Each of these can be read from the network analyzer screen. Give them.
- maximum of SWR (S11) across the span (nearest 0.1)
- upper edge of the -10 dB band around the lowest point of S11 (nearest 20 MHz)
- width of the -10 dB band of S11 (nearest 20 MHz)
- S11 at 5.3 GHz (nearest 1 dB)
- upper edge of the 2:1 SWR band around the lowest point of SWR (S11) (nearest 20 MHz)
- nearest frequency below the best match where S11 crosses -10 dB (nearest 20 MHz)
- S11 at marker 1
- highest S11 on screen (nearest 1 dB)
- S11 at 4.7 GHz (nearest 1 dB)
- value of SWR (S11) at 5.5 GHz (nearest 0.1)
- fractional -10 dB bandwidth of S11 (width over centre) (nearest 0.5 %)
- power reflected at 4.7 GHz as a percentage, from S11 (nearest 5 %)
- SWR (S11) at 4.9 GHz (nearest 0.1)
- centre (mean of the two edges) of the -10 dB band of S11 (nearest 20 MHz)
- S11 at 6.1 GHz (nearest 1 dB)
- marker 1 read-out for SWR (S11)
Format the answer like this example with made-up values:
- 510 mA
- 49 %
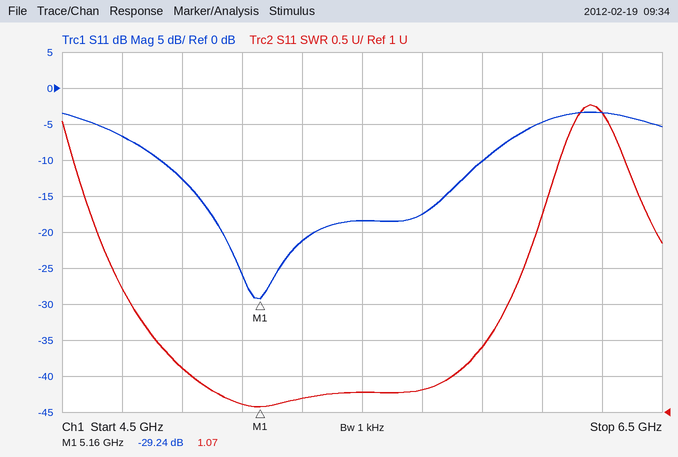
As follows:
- 5.3
- 5.90 GHz
- 1.08 GHz
- -21 dB
- 5.92 GHz
- 4.82 GHz
- -29.24 dB
- -3 dB
- -7 dB
- 1.3
- 20.0 %
- 20 %
- 1.6
- 5.36 GHz
- -5 dB
- 1.07
